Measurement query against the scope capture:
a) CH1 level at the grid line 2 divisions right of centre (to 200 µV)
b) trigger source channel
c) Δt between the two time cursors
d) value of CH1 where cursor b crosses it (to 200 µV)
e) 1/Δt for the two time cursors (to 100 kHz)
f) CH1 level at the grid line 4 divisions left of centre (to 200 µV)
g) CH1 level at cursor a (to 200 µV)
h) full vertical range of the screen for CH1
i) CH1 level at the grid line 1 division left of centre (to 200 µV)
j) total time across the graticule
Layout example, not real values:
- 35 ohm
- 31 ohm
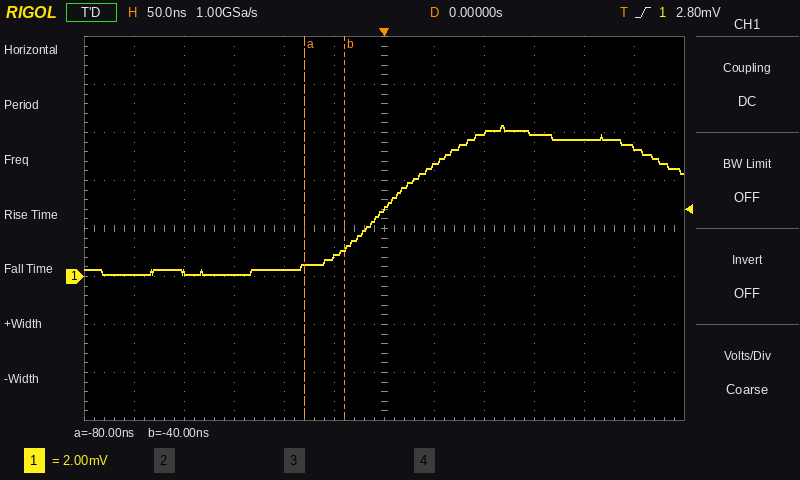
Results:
- 6.0 mV
- CH1
- 40 ns
- 1.2 mV
- 25.0 MHz
- 200 µV
- 400 µV
- 16 mV
- 800 µV
- 600 ns
